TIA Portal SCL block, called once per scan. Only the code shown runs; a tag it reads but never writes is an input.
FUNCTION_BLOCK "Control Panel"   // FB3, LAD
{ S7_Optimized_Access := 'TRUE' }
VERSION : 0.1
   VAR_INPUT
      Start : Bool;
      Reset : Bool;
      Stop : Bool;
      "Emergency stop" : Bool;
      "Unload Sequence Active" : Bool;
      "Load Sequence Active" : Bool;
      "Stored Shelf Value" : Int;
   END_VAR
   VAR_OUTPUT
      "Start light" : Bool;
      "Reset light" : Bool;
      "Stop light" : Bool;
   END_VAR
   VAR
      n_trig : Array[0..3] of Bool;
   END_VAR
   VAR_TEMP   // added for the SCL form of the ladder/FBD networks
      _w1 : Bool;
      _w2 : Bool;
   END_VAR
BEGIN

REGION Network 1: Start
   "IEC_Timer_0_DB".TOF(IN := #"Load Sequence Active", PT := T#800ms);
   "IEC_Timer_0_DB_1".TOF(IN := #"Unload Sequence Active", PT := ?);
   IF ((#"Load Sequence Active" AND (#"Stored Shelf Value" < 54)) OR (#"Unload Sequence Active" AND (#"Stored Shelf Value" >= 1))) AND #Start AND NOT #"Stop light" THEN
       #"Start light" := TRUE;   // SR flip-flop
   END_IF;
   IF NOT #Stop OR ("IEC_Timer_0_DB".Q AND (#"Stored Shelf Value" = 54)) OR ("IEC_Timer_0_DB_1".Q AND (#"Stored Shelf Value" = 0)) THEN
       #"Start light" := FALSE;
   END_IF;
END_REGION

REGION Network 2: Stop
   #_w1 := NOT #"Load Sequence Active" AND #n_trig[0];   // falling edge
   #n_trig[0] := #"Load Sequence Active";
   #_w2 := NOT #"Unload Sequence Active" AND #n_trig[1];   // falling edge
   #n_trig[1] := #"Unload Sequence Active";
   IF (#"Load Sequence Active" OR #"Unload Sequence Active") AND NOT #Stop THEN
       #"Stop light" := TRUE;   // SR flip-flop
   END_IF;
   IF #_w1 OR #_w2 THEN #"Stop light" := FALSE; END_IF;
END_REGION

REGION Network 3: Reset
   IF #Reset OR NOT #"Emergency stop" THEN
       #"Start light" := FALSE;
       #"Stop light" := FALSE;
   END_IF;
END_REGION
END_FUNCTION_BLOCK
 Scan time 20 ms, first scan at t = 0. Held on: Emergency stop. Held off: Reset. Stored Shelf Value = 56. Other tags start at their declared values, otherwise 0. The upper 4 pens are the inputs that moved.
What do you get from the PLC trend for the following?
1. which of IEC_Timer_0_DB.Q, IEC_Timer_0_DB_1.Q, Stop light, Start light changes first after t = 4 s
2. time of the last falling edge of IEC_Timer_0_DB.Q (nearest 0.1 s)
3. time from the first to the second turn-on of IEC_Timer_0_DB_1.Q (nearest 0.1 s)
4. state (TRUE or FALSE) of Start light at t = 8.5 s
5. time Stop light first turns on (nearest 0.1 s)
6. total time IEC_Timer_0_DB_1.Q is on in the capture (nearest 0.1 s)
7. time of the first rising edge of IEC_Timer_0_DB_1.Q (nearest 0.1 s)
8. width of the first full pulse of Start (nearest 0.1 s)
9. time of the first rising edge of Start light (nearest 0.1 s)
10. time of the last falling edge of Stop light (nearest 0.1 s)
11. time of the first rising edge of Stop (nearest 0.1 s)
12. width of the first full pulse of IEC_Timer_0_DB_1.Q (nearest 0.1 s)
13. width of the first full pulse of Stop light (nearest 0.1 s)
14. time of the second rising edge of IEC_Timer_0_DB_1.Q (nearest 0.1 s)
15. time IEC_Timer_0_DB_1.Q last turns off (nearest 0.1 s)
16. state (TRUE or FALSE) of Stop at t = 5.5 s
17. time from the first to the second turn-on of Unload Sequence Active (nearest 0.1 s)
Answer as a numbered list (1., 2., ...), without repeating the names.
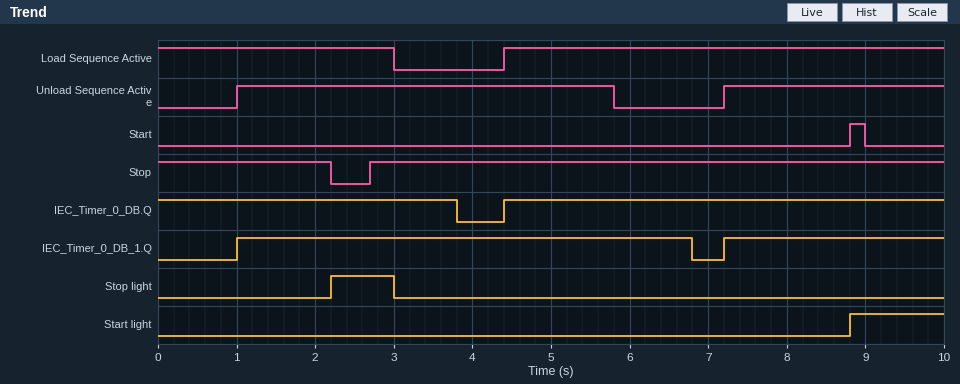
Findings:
1. IEC_Timer_0_DB.Q
2. 3.8 s
3. 6.2 s
4. FALSE
5. 2.2 s
6. 8.6 s
7. 1.0 s
8. 0.2 s
9. 8.8 s
10. 3.0 s
11. 2.7 s
12. 5.8 s
13. 0.8 s
14. 7.2 s
15. 6.8 s
16. TRUE
17. 6.2 s
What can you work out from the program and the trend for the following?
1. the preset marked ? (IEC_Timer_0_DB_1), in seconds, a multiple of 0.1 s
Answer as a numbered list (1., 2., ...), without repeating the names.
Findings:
1. 1.0 s
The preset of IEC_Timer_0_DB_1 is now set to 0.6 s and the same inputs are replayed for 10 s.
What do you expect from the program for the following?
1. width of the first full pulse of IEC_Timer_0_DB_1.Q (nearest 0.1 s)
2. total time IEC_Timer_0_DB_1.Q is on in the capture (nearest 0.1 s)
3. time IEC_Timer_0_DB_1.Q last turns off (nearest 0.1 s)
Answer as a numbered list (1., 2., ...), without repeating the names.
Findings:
1. 5.4 s
2. 8.2 s
3. 6.4 s
